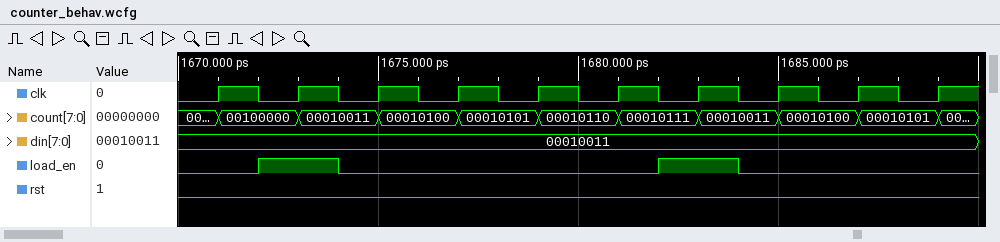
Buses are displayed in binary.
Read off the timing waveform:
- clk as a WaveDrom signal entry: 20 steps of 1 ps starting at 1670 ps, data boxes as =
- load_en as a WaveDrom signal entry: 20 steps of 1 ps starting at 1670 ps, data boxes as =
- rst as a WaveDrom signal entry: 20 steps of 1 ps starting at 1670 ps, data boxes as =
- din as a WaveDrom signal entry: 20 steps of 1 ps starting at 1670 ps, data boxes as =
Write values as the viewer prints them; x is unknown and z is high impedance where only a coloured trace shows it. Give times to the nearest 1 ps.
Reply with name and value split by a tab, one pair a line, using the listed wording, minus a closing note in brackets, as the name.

clk as a WaveDrom signal entry: 20 steps of 1 ps starting at 1670 ps, data boxes as =	{name: 'clk', wave: '01010101010101010101'}
load_en as a WaveDrom signal entry: 20 steps of 1 ps starting at 1670 ps, data boxes as =	{name: 'load_en', wave: '0.1.0.......1.0.....'}
rst as a WaveDrom signal entry: 20 steps of 1 ps starting at 1670 ps, data boxes as =	{name: 'rst', wave: '0...................'}
din as a WaveDrom signal entry: 20 steps of 1 ps starting at 1670 ps, data boxes as =	{name: 'din', wave: '=...................', data: '00010011'}
